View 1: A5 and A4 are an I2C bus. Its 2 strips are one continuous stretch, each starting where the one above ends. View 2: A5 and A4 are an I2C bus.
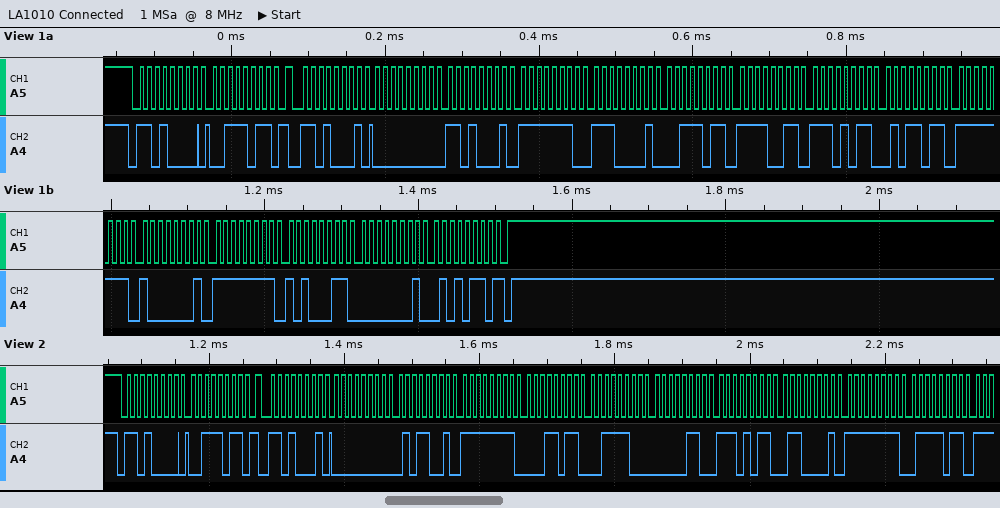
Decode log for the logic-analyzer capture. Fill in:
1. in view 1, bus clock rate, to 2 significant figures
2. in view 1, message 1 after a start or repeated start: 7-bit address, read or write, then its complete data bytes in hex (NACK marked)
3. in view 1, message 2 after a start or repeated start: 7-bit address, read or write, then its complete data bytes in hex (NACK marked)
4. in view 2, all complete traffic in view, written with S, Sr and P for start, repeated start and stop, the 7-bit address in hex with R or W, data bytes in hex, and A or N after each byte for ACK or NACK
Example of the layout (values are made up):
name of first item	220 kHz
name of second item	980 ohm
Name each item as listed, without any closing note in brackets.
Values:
in view 1, bus clock rate, to 2 significant figures	100 kHz
in view 1, message 1 after a start or repeated start: 7-bit address, read or write, then its complete data bytes in hex	0x68 write: 3B
in view 1, message 2 after a start or repeated start: 7-bit address, read or write, then its complete data bytes in hex	0x68 read: 00 D1 FE E1 3B F3 EB 5B FF 81 FF A3 01 56 NACK
in view 2, all complete traffic in view, written with S, Sr and P for start, repeated start and stop, the 7-bit address in hex with R or W, data bytes in hex, and A or N after each byte for ACK or NACK	S 68W A 3B A Sr 68R A 00 A 59 A FF A 1B A 3C A 06 A EB A 61 A FF A 7B A
